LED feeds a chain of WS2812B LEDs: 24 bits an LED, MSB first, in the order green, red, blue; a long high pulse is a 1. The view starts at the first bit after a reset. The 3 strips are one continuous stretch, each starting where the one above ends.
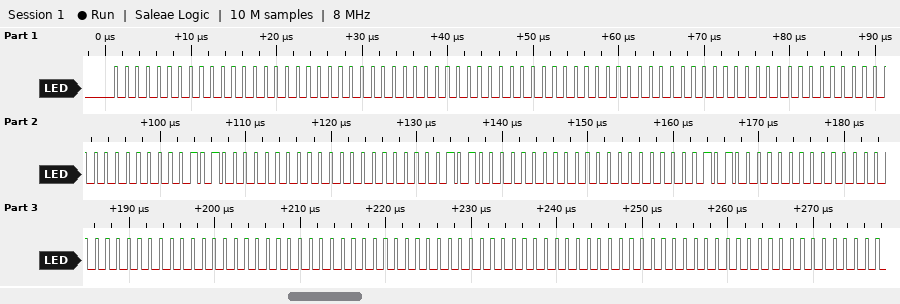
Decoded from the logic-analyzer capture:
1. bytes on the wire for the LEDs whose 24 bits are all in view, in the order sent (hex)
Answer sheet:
00 00 00 00 00 00 00 00 00 00 28 00 00 28 00 00 28 00 00 00 00 00 00 00 00 00 00
